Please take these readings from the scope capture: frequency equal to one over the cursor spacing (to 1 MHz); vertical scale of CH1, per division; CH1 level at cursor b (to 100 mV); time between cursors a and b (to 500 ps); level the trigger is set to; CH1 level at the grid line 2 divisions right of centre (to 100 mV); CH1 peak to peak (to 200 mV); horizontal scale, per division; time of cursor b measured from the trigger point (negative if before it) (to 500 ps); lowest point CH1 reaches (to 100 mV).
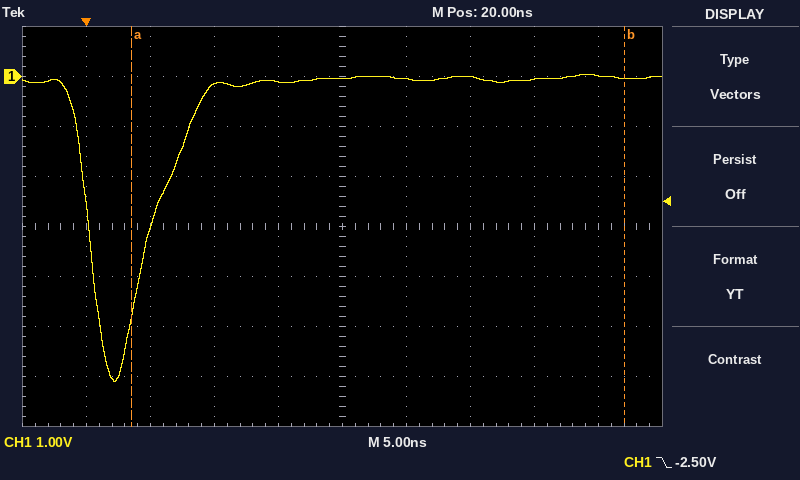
26 MHz
1 V
0.0 V
38.5 ns
-2.50 V
0.0 V
6.2 V
5 ns
+42.0 ns
-6.1 V
